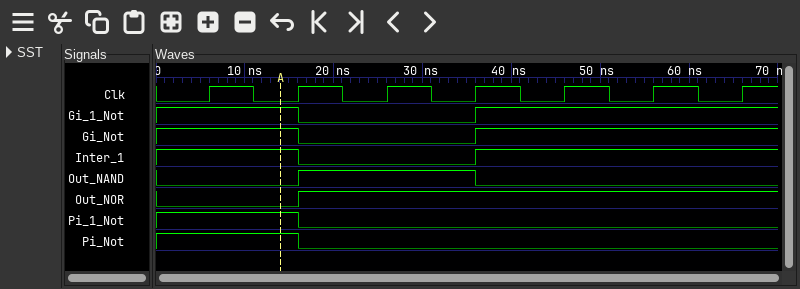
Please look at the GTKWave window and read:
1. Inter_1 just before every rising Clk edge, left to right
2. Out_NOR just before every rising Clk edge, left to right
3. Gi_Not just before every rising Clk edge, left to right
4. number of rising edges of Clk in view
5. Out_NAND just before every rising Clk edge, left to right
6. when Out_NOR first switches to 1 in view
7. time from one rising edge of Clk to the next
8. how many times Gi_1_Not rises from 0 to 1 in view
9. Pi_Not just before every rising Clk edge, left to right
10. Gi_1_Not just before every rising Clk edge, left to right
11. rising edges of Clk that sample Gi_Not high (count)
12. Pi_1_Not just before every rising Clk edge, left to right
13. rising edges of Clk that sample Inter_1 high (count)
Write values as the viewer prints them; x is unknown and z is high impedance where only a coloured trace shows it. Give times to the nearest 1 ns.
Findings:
1 1 0 0 1 1 1
0 0 1 1 1 1 1
1 1 0 0 1 1 1
7
0 0 1 1 0 0 0
16 ns
10 ns
1
1 1 0 0 0 0 0
1 1 0 0 1 1 1
5
1 1 0 0 0 0 0
5
